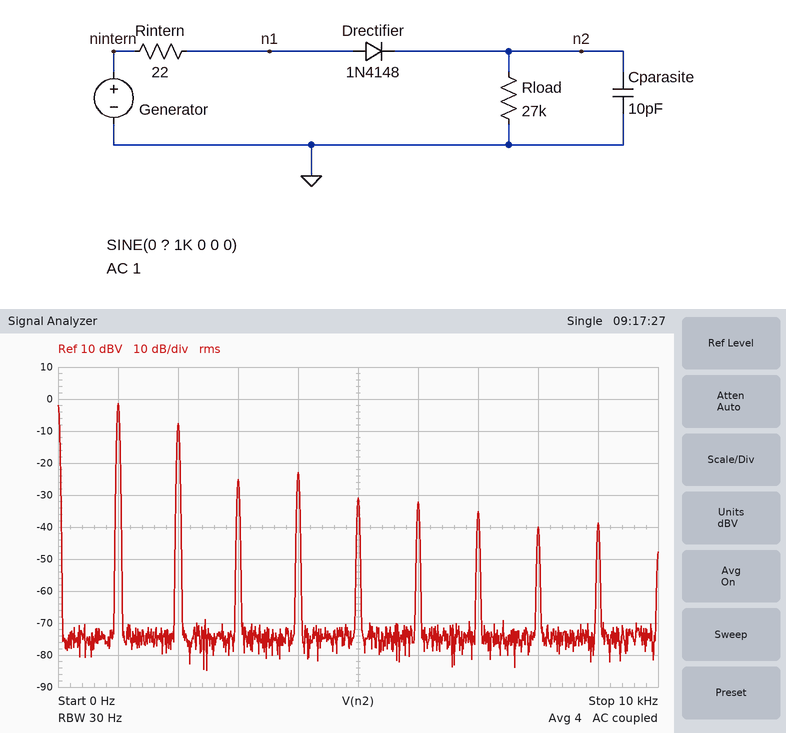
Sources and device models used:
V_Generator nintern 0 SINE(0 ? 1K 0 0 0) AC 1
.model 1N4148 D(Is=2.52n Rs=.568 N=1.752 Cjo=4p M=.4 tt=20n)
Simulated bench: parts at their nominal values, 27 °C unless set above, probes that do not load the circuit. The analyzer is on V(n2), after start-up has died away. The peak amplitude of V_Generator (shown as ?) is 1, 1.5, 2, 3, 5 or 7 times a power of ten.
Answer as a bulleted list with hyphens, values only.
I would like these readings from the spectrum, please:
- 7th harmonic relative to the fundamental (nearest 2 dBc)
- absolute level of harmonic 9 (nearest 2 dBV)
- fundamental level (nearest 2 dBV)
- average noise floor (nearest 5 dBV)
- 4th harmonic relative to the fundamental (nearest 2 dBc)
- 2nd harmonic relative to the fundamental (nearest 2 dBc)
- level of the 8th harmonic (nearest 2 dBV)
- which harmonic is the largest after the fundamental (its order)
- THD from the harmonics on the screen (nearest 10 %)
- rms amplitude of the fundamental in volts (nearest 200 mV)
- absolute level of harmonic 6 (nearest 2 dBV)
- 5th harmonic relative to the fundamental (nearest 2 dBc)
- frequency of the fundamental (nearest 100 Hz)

- -34 dBc
- -38 dBV
- -2 dBV
- -75 dBV
- -22 dBc
- -6 dBc
- -40 dBV
- 2
- 50 %
- 800 mV
- -32 dBV
- -30 dBc
- 1.0 kHz
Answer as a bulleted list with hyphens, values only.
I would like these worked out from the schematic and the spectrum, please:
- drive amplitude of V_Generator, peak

- 3 V
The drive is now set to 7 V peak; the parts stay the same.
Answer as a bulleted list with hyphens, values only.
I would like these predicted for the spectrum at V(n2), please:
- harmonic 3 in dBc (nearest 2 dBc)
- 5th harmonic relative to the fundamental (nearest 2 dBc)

- -30 dBc
- -36 dBc
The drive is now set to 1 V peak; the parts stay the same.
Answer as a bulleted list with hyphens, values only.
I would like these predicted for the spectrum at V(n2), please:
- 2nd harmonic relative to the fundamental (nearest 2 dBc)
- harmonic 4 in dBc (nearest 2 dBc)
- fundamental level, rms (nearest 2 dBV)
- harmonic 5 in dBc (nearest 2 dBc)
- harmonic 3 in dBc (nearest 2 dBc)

- -4 dBc
- -30 dBc
- -14 dBV
- -24 dBc
- -14 dBc
